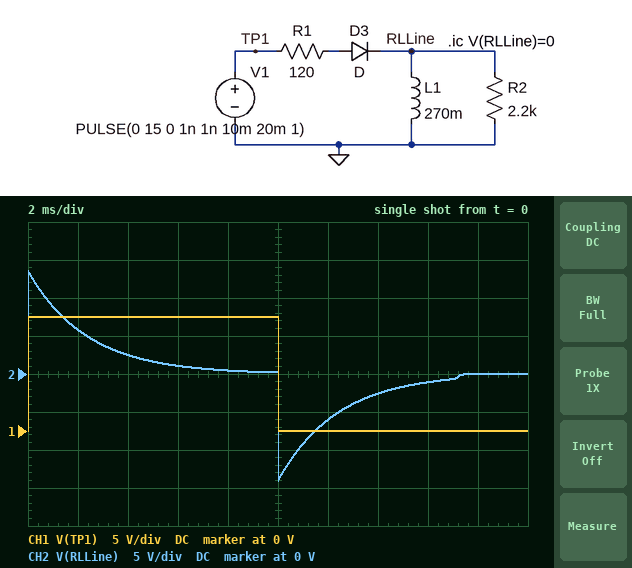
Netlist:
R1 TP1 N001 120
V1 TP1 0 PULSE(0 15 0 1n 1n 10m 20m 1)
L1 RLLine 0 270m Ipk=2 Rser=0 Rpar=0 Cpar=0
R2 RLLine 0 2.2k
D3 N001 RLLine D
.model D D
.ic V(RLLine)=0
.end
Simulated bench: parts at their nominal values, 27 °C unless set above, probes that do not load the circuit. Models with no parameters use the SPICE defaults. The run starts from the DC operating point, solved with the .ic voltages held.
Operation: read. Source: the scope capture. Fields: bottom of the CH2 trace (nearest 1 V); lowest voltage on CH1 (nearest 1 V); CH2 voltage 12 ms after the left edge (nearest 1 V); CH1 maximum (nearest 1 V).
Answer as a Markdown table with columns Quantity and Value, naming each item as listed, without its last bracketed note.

| Quantity | Value |
|---|---|
| bottom of the CH2 trace | -14 V |
| lowest voltage on CH1 | 0 V |
| CH2 voltage 12 ms after the left edge | -6 V |
| CH1 maximum | 15 V |
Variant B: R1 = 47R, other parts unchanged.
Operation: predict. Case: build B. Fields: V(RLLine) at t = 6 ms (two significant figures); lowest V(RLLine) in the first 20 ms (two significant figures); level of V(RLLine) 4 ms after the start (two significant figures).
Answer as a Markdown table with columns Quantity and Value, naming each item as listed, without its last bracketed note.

| Quantity | Value |
|---|---|
| V(RLLine) at t = 6 ms | 5.0 V |
| lowest V(RLLine) in the first 20 ms | -12 V |
| level of V(RLLine) 4 ms after the start | 7.0 V |
